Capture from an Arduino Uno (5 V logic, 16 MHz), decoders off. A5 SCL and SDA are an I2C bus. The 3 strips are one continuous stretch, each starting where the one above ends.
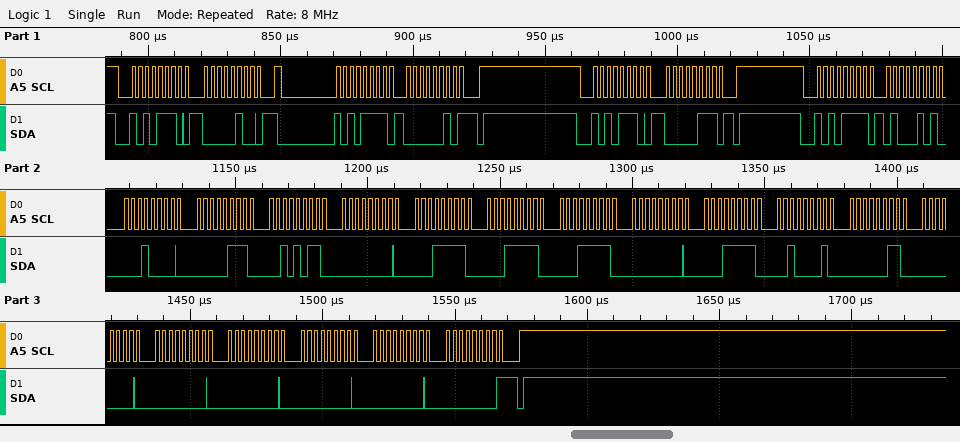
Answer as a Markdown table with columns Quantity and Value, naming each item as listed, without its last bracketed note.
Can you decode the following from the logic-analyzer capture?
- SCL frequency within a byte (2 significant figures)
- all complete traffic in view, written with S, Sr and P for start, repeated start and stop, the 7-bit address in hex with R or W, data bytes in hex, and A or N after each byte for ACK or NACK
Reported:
| Quantity | Value |
|---|---|
| SCL frequency within a byte | 400 kHz |
| all complete traffic in view, written with S, Sr and P for start, repeated start and stop, the 7-bit address in hex with R or W, data bytes in hex, and A or N after each byte for ACK or NACK | S 57W A 04 A Sr 57R A 02 N P S 57W A 07 A P S 57R A 45 A 10 A 07 A 2B A 00 A 1F A 1F A 1F A 00 A 1F A 21 A 03 A 00 A 00 A 00 A 00 A 00 A 00 N P |
